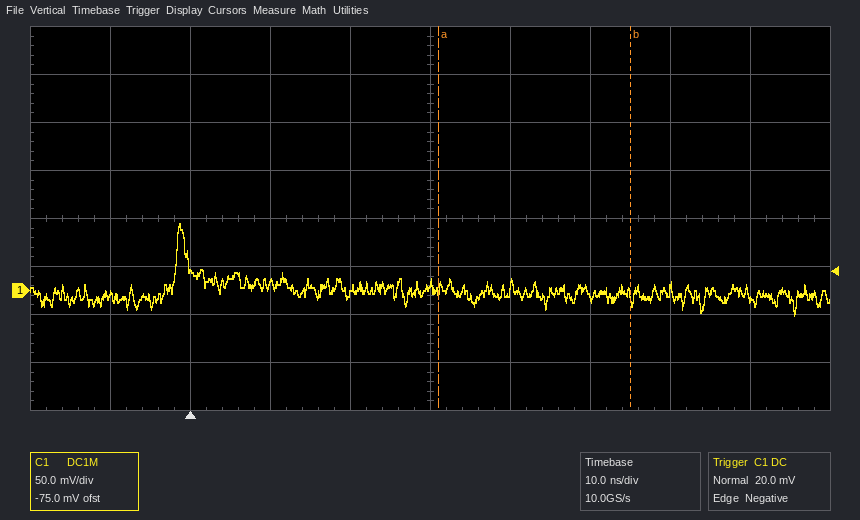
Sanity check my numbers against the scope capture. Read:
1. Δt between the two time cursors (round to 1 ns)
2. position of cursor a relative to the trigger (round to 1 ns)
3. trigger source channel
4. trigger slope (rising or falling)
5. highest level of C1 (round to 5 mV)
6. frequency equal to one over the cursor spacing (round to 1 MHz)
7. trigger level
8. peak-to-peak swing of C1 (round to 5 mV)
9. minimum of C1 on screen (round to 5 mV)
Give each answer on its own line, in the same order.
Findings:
24 ns
+31 ns
C1
falling
70 mV
42 MHz
20.0 mV
95 mV
-25 mV
